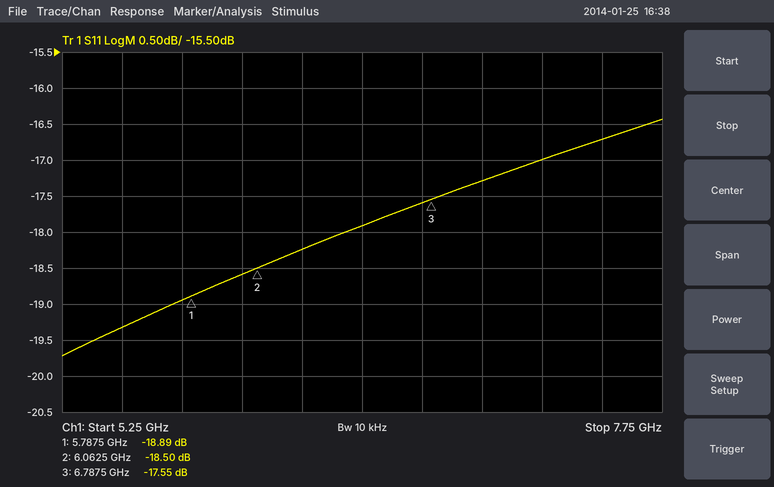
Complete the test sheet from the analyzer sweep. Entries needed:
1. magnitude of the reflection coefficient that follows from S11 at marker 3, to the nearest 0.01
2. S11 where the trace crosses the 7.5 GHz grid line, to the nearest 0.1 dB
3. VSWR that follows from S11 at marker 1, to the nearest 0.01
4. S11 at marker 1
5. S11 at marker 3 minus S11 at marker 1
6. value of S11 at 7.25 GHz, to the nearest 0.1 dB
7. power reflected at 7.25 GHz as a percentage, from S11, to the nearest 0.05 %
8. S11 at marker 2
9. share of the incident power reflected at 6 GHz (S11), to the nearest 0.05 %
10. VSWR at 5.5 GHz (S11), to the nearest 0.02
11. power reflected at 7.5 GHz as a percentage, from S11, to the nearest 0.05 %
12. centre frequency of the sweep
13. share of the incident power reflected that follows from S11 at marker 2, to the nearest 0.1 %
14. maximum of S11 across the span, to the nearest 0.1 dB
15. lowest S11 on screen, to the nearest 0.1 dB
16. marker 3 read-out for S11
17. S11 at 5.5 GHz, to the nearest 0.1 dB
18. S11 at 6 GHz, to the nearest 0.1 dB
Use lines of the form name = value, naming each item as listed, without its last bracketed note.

magnitude of the reflection coefficient that follows from S11 at marker 3, to the nearest 0.01 = 0.13
S11 where the trace crosses the 7.5 GHz grid line, to the nearest 0.1 dB = -16.7 dB
VSWR that follows from S11 at marker 1, to the nearest 0.01 = 1.26
S11 at marker 1 = -18.89 dB
S11 at marker 3 minus S11 at marker 1 = 1.34 dB
value of S11 at 7.25 GHz, to the nearest 0.1 dB = -17.0 dB
power reflected at 7.25 GHz as a percentage, from S11, to the nearest 0.05 % = 2.00 %
S11 at marker 2 = -18.50 dB
share of the incident power reflected at 6 GHz (S11), to the nearest 0.05 % = 1.40 %
VSWR at 5.5 GHz (S11), to the nearest 0.02 = 1.24
power reflected at 7.5 GHz as a percentage, from S11, to the nearest 0.05 % = 2.15 %
centre frequency of the sweep = 6.5 GHz
share of the incident power reflected that follows from S11 at marker 2, to the nearest 0.1 % = 1.4 %
maximum of S11 across the span, to the nearest 0.1 dB = -16.4 dB
lowest S11 on screen, to the nearest 0.1 dB = -19.7 dB
marker 3 read-out for S11 = -17.55 dB
S11 at 5.5 GHz, to the nearest 0.1 dB = -19.3 dB
S11 at 6 GHz, to the nearest 0.1 dB = -18.6 dB
